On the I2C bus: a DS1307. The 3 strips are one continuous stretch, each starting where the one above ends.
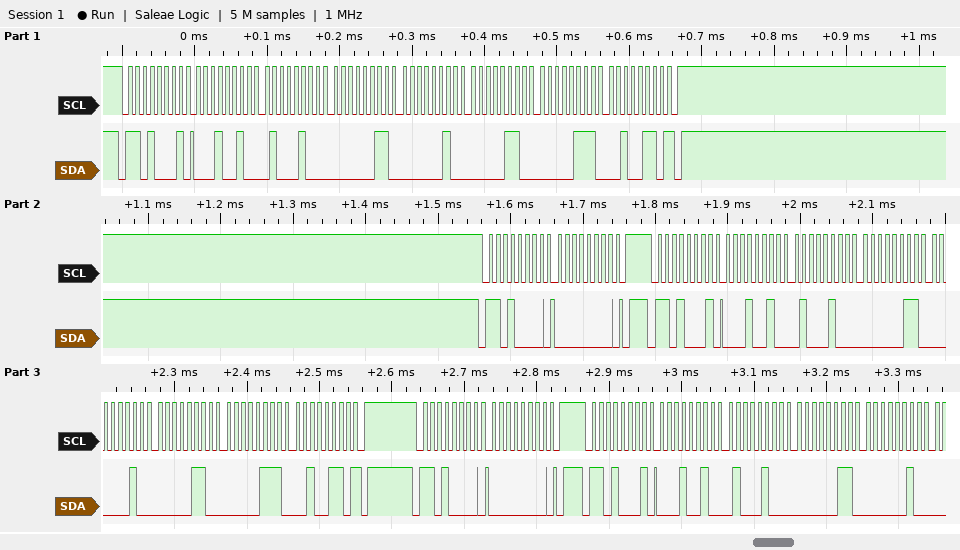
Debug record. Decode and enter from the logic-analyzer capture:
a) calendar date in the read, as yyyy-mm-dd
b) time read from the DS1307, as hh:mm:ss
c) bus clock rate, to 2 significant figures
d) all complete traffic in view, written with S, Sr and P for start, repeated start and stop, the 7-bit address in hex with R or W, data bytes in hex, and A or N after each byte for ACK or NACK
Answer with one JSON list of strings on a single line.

["2026-07-06", "03:44:12", "100 kHz", "S 68R A 12 A 44 A 03 A 02 A 06 A 07 A 26 N P S 68W A 00 A P S 68R A 12 A 44 A 03 A 02 A 06 A 07 A 26 N P S 68W A 00 A P S 68R A 12 A 44 A 03 A 02 A"]
